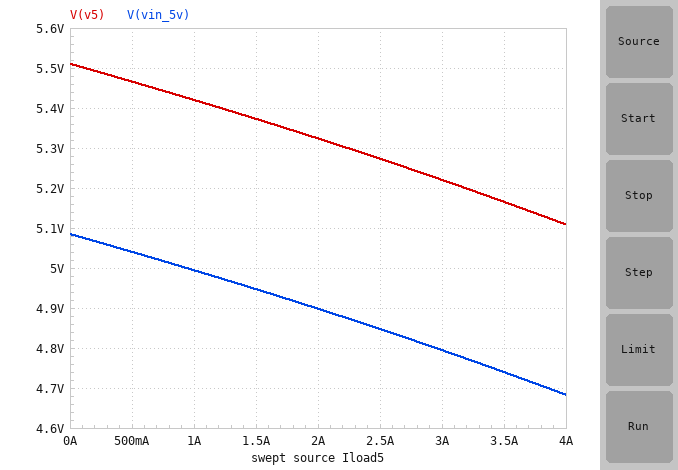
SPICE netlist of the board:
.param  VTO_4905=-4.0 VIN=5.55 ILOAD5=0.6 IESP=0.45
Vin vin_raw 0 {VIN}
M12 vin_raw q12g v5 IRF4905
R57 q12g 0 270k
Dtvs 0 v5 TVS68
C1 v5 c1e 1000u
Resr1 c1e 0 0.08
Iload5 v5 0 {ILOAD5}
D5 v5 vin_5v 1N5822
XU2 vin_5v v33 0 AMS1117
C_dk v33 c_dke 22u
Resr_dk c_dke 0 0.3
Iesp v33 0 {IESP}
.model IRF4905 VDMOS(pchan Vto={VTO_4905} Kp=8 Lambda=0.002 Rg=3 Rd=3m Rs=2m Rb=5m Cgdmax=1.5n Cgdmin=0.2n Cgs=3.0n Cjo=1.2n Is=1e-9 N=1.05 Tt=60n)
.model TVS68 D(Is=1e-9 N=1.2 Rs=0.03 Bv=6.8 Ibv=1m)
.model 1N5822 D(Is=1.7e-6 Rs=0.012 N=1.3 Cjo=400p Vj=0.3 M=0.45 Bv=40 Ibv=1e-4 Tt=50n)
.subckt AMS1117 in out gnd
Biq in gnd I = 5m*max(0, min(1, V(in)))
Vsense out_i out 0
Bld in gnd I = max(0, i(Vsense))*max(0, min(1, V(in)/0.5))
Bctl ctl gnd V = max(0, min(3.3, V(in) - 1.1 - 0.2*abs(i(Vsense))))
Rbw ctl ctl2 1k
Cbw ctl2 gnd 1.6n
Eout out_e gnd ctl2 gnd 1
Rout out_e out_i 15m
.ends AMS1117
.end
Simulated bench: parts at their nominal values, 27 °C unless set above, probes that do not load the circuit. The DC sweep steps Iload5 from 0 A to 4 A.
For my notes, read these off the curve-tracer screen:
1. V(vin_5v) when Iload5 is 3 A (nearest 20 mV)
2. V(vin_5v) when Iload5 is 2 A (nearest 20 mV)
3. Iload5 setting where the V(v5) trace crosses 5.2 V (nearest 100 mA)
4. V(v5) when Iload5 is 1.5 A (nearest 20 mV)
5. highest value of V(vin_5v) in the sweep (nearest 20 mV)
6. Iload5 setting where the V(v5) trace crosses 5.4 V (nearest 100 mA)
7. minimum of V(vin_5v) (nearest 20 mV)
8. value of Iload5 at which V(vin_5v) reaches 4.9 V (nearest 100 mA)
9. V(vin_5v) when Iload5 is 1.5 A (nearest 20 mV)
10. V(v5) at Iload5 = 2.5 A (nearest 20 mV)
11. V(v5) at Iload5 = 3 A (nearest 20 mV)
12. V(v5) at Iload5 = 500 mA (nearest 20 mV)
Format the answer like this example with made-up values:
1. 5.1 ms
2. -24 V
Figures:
1. 4.80 V
2. 4.90 V
3. 3.2 A
4. 5.38 V
5. 5.08 V
6. 1.2 A
7. 4.68 V
8. 2.0 A
9. 4.94 V
10. 5.28 V
11. 5.22 V
12. 5.46 V
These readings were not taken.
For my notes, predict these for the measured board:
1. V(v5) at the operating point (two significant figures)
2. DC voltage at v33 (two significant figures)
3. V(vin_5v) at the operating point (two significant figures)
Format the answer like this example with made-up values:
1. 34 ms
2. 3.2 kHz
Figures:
1. 5.5 V
2. 3.3 V
3. 5.0 V
